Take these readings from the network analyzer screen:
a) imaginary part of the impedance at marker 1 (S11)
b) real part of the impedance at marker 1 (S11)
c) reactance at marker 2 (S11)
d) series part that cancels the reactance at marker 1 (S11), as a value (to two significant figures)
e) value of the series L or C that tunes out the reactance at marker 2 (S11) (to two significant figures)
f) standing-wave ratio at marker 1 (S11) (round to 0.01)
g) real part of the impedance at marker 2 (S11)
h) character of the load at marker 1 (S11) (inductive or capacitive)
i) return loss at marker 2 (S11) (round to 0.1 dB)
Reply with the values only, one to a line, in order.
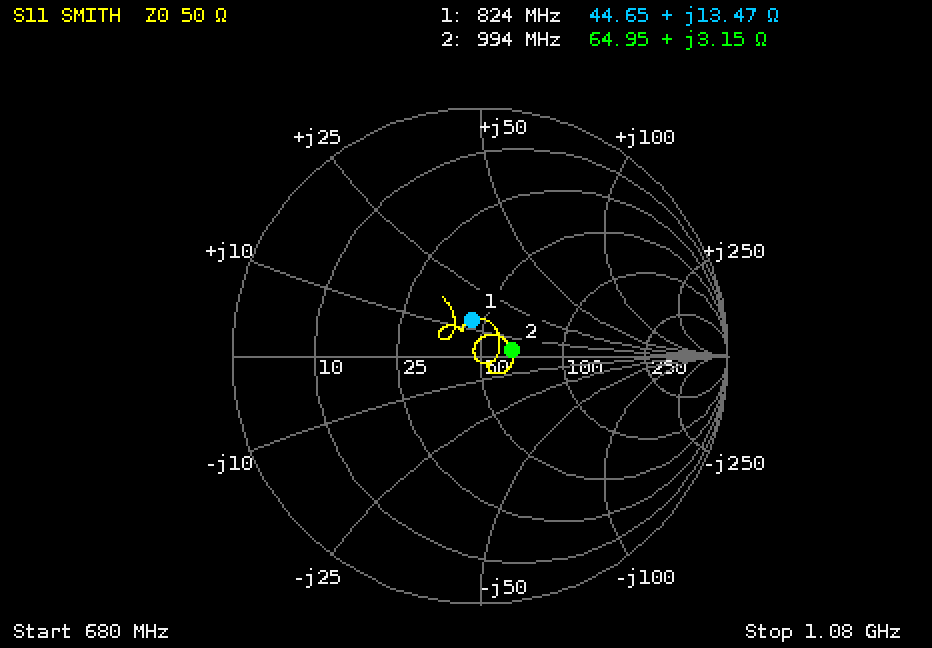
+13.47 Ω
44.65 Ω
+3.15 Ω
14 pF
51 pF
1.36
64.95 Ω
inductive
17.5 dB
